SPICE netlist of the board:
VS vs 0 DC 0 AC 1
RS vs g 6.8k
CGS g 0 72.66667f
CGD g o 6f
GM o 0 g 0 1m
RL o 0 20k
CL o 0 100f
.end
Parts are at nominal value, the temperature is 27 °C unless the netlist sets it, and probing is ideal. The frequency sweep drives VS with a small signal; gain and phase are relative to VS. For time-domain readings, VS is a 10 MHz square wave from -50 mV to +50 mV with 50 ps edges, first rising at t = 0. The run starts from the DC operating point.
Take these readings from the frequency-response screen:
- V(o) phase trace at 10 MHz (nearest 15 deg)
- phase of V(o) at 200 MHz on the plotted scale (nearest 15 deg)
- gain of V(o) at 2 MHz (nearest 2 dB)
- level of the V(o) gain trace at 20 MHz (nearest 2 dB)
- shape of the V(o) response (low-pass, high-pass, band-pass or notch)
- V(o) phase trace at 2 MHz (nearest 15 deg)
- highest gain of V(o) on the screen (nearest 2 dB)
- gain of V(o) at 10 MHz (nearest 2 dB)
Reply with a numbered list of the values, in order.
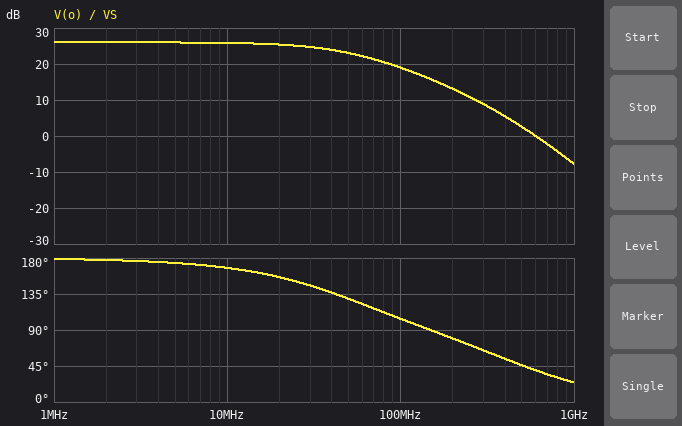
1. 165 deg
2. 75 deg
3. 26 dB
4. 26 dB
5. low-pass
6. 180 deg
7. 26 dB
8. 26 dB
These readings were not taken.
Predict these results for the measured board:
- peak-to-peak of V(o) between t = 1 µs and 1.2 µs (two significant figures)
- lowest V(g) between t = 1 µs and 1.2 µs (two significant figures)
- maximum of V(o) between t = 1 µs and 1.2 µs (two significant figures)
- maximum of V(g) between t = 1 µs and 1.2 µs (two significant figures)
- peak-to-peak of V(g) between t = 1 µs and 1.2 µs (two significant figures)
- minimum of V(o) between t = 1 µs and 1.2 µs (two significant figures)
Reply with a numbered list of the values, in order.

1. 2.0 V
2. -50 mV
3. 1.0 V
4. 50 mV
5. 100 mV
6. -1.0 V
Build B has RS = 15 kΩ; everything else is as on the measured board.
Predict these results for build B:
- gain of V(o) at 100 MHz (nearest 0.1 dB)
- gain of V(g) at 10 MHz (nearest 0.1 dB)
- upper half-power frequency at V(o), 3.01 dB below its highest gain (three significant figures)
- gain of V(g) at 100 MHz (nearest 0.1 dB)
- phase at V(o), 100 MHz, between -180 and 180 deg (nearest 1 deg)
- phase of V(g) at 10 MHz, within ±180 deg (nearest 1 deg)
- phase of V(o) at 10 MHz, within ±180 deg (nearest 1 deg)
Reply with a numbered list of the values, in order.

1. 15.9 dB
2. -0.3 dB
3. 34.5 MHz
4. -5.7 dB
5. 90 deg
6. -10 deg
7. 162 deg
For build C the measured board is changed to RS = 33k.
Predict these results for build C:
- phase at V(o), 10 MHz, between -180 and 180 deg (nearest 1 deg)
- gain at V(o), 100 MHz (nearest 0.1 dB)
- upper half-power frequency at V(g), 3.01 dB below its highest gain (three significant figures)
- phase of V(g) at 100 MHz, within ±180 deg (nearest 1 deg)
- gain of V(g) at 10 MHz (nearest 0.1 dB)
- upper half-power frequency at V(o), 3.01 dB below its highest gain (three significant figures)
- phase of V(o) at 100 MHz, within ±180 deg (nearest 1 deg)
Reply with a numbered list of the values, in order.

1. 151 deg
2. 11.1 dB
3. 21.3 MHz
4. -49 deg
5. -0.9 dB
6. 19.8 MHz
7. 78 deg
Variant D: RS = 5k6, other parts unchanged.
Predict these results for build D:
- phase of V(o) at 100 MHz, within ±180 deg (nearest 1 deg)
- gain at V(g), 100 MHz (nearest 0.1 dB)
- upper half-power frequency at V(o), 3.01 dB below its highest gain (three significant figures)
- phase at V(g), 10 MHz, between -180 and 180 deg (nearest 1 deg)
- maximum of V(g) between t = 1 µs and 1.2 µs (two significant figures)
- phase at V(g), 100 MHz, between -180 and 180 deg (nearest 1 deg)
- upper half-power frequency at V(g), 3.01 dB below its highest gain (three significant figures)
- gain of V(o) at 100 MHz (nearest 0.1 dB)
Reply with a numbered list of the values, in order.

1. 107 deg
2. -2.1 dB
3. 54.0 MHz
4. -4 deg
5. 50 mV
6. -20 deg
7. 184 MHz
8. 19.5 dB
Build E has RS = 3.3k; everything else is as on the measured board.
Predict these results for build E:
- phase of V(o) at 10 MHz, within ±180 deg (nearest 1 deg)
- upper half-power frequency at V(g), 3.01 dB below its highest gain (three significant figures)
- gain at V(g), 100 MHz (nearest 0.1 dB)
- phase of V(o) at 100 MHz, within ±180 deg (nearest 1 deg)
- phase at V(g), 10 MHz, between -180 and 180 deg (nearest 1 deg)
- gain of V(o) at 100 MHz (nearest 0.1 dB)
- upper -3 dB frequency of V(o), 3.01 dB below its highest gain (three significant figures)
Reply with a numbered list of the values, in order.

1. 170 deg
2. 459 MHz
3. -1.2 dB
4. 114 deg
5. -2 deg
6. 20.4 dB
7. 61.7 MHz
